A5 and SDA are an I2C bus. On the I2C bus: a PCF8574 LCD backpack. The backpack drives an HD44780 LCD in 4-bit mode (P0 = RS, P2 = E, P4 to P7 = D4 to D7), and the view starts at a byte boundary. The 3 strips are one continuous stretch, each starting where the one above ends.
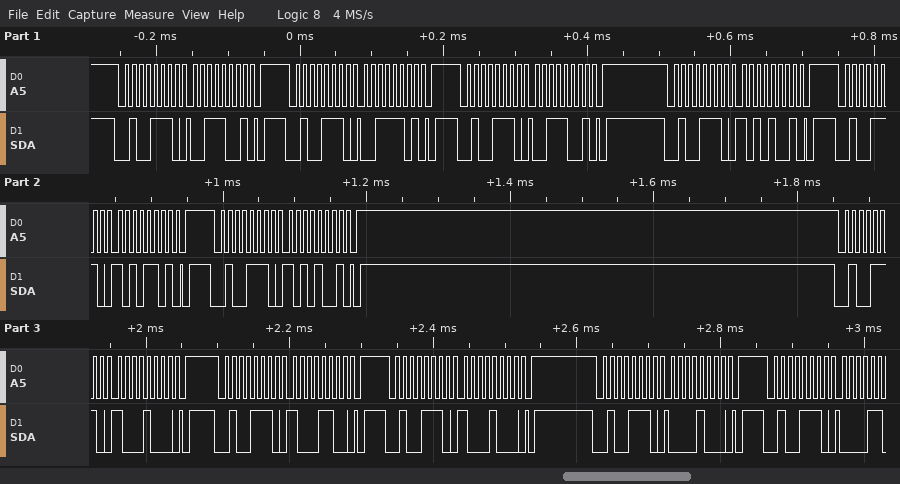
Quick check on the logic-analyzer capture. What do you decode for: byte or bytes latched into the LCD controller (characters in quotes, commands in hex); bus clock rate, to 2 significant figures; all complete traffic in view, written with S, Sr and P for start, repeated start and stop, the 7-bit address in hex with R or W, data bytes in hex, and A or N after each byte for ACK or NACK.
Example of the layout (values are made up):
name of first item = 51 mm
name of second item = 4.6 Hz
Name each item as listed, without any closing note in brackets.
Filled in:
byte or bytes latched into the LCD controller = ':'
bus clock rate, to 2 significant figures = 100 kHz
all complete traffic in view, written with S, Sr and P for start, repeated start and stop, the 7-bit address in hex with R or W, data bytes in hex, and A or N after each byte for ACK or NACK = S 27W A 39 A P S 27W A 3D A P S 27W A 39 A P S 27W A A9 A P S 27W A AD A P S 27W A A9 A P S 27W A 88 A P S 27W A 8C A P S 27W A 88 A P S 27W A 08 A P S 27W A
